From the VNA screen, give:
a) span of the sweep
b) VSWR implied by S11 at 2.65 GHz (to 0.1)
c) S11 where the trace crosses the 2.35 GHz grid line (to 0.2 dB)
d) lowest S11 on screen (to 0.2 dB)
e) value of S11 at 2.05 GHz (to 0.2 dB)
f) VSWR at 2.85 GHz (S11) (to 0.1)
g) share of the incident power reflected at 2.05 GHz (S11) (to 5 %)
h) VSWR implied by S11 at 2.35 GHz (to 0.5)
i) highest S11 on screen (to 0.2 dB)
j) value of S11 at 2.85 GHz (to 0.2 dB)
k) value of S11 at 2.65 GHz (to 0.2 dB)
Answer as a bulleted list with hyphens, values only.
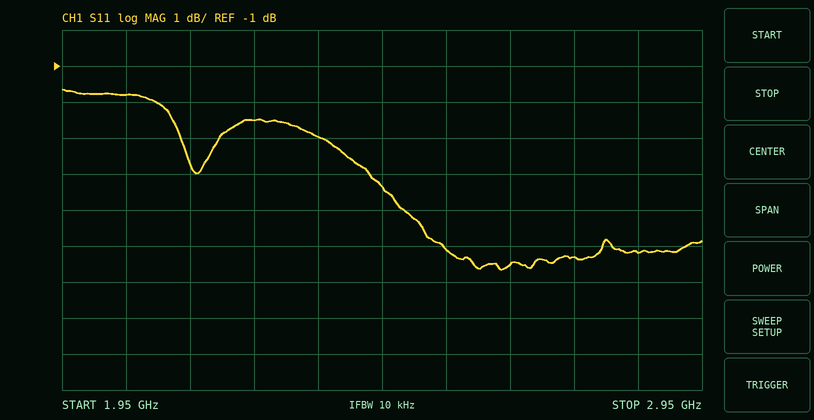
- 1 GHz
- 2.8
- -3.0 dB
- -6.6 dB
- -1.8 dB
- 2.9
- 65 %
- 6.0
- -1.6 dB
- -6.2 dB
- -6.6 dB
